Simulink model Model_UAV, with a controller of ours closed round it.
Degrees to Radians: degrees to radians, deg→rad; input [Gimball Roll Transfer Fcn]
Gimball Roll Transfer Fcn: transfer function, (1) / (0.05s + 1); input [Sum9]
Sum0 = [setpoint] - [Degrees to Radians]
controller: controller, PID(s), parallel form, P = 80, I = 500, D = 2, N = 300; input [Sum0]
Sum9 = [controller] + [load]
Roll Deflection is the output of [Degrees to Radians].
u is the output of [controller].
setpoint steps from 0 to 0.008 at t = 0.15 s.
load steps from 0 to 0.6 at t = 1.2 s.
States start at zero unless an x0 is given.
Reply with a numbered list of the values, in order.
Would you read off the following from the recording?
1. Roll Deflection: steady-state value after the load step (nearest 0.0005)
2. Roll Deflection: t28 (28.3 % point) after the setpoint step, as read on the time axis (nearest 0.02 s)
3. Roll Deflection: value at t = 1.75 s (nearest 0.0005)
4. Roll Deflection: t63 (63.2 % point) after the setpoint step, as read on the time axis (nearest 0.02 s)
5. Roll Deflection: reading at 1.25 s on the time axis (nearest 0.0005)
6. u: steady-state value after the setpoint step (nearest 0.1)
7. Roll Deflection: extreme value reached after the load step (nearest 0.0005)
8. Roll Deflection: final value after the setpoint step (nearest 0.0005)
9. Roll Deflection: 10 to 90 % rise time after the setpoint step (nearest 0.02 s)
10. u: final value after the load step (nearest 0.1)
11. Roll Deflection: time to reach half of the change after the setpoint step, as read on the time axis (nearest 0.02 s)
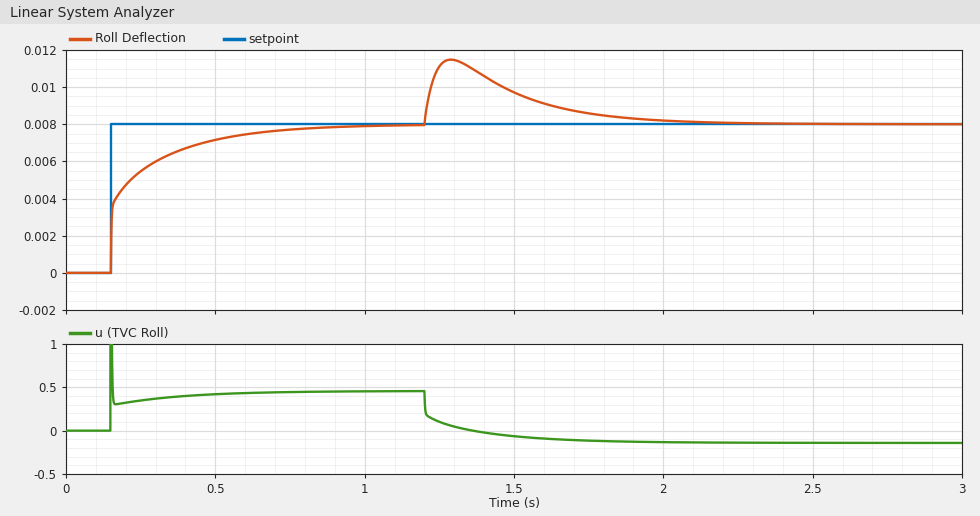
1. 0.0080
2. 0.16 s
3. 0.0085
4. 0.22 s
5. 0.0110
6. 0.5
7. 0.0115
8. 0.0080
9. 0.36 s
10. -0.1
11. 0.16 s
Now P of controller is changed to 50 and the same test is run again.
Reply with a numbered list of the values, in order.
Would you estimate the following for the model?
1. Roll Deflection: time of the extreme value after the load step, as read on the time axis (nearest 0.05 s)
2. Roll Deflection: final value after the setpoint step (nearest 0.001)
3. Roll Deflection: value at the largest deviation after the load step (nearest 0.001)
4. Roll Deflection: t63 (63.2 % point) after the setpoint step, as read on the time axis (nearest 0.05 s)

1. 1.30 s
2. 0.008
3. 0.012
4. 0.25 s
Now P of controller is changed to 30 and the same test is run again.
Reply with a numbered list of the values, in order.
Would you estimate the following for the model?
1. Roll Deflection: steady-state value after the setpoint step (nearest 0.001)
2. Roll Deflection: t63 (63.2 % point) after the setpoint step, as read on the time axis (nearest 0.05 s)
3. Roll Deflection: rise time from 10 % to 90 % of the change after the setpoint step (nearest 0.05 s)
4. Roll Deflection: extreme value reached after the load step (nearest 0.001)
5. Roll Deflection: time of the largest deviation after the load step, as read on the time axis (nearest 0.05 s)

1. 0.008
2. 0.30 s
3. 0.30 s
4. 0.013
5. 1.30 s
